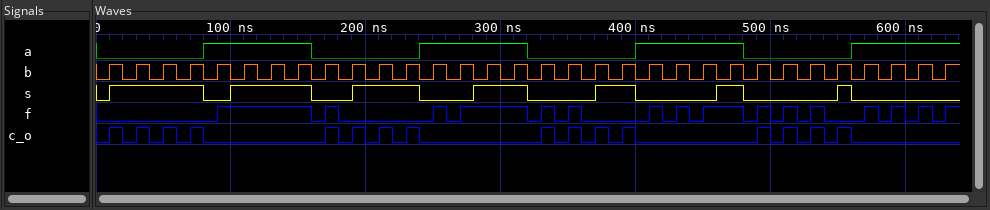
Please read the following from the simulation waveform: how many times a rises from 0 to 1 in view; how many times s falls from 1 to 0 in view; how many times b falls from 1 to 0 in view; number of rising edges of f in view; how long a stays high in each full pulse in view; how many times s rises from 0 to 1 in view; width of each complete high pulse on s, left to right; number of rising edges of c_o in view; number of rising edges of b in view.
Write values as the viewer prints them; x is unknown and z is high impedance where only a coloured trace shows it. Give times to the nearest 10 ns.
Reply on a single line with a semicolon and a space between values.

4; 7; 31; 16; 80 ns, 80 ns, 80 ns; 7; 70 ns, 60 ns, 50 ns, 40 ns, 30 ns, 20 ns, 10 ns; 16; 32
